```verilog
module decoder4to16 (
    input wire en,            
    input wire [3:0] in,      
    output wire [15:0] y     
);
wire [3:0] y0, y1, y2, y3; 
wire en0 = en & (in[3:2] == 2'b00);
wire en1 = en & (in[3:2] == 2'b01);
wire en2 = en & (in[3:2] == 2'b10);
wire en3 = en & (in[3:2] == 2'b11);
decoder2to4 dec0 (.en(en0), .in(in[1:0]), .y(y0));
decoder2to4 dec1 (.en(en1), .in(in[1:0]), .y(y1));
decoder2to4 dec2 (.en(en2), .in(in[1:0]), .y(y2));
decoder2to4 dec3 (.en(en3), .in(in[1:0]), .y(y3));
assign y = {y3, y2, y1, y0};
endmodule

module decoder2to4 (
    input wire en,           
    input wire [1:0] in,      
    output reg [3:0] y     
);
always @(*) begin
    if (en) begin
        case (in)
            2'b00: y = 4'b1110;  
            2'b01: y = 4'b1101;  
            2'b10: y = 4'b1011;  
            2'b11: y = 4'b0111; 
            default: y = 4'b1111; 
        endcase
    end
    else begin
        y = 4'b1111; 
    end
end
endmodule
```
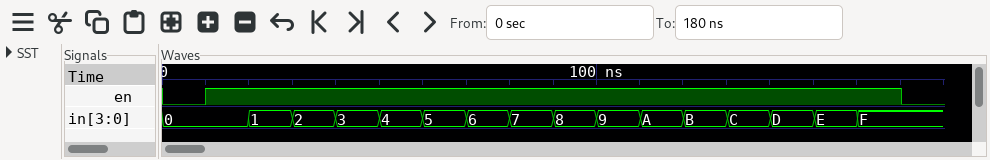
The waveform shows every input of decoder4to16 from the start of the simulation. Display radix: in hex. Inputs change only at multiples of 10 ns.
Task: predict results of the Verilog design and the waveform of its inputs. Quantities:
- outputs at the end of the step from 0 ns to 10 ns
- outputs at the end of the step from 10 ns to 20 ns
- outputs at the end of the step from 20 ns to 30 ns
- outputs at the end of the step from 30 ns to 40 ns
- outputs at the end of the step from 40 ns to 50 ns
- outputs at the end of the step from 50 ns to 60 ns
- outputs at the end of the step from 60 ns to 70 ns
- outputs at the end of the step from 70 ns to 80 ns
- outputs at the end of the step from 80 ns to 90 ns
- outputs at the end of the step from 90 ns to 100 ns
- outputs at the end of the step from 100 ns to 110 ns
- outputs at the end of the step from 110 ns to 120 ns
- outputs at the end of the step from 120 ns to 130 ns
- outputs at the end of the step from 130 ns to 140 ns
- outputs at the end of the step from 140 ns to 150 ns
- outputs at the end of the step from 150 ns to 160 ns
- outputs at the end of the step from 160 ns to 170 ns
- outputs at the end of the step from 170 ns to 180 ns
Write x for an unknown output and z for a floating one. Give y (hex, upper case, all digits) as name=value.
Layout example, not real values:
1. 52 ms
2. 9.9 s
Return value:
1. y=FFFF
2. y=FFFE
3. y=FFFD
4. y=FFFB
5. y=FFF7
6. y=FFEF
7. y=FFDF
8. y=FFBF
9. y=FF7F
10. y=FEFF
11. y=FDFF
12. y=FBFF
13. y=F7FF
14. y=EFFF
15. y=DFFF
16. y=BFFF
17. y=7FFF
18. y=FFFF
